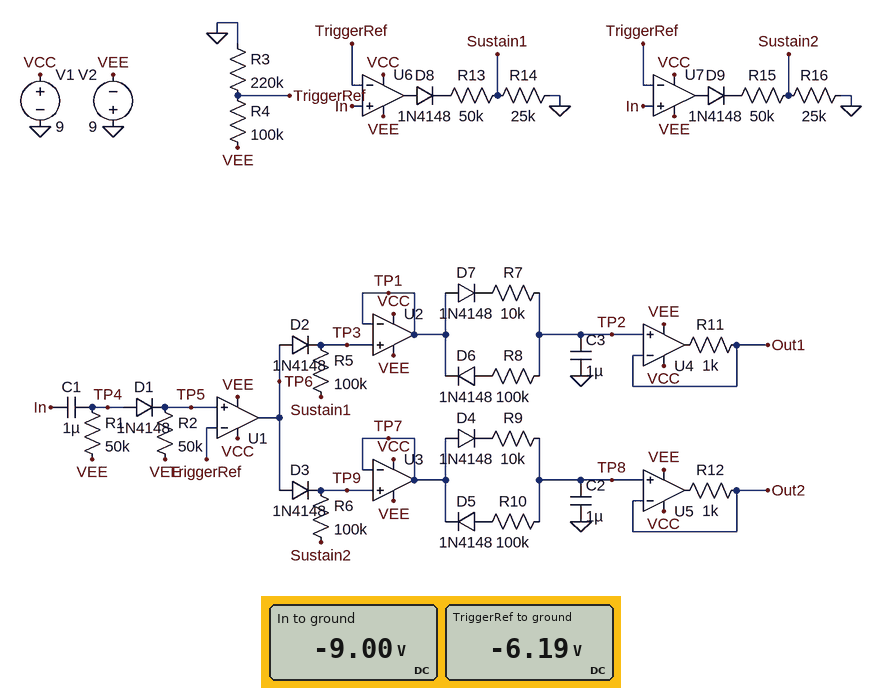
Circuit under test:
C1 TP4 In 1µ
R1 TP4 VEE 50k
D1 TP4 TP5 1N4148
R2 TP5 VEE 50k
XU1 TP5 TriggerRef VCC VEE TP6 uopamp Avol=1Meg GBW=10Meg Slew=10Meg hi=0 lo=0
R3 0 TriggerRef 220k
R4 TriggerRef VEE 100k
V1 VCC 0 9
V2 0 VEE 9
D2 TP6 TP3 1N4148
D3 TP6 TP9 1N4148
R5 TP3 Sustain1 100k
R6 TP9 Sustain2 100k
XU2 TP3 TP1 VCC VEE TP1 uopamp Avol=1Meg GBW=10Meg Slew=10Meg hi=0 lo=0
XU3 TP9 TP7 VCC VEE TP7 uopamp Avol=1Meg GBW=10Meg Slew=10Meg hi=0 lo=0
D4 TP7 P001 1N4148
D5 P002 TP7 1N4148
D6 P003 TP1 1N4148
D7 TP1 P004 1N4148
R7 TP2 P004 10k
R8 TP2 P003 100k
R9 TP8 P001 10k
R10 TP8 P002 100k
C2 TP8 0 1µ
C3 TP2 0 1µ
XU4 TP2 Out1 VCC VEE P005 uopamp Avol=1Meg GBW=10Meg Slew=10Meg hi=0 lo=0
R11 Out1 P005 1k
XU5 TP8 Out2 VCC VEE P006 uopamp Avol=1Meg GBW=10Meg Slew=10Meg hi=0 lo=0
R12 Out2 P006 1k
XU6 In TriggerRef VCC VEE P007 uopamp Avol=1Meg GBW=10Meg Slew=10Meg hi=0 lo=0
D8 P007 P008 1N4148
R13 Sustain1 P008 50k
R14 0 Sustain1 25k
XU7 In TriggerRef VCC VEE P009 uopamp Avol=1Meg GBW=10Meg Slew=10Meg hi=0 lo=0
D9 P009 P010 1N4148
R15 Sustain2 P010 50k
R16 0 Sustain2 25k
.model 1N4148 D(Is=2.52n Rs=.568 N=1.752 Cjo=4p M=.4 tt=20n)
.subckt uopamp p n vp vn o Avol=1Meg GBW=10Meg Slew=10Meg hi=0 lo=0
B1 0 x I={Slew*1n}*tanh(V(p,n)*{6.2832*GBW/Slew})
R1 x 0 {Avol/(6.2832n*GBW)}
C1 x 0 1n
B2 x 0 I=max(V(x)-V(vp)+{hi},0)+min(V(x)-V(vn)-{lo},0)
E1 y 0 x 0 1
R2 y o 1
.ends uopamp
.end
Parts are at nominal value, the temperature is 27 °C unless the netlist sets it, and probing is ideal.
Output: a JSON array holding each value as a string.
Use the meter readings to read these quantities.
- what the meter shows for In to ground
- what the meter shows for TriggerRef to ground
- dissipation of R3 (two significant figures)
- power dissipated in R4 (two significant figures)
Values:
["-9.00 V", "-6.19 V", "170 µW", "79 µW"]
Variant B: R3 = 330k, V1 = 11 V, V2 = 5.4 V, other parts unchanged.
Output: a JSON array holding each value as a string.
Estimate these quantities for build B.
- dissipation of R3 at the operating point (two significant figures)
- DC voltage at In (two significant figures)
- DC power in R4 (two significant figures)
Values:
["52 µW", "-5.4 V", "16 µW"]
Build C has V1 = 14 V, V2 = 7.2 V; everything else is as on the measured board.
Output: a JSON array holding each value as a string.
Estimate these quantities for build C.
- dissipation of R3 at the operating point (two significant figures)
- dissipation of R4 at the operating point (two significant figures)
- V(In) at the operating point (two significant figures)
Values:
["110 µW", "51 µW", "-7.2 V"]
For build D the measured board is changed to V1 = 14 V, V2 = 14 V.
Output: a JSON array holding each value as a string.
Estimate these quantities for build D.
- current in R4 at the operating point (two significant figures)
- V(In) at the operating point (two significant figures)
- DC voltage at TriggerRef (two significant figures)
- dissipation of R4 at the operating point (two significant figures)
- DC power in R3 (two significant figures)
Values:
["44 µA", "-14 V", "-9.6 V", "190 µW", "420 µW"]
